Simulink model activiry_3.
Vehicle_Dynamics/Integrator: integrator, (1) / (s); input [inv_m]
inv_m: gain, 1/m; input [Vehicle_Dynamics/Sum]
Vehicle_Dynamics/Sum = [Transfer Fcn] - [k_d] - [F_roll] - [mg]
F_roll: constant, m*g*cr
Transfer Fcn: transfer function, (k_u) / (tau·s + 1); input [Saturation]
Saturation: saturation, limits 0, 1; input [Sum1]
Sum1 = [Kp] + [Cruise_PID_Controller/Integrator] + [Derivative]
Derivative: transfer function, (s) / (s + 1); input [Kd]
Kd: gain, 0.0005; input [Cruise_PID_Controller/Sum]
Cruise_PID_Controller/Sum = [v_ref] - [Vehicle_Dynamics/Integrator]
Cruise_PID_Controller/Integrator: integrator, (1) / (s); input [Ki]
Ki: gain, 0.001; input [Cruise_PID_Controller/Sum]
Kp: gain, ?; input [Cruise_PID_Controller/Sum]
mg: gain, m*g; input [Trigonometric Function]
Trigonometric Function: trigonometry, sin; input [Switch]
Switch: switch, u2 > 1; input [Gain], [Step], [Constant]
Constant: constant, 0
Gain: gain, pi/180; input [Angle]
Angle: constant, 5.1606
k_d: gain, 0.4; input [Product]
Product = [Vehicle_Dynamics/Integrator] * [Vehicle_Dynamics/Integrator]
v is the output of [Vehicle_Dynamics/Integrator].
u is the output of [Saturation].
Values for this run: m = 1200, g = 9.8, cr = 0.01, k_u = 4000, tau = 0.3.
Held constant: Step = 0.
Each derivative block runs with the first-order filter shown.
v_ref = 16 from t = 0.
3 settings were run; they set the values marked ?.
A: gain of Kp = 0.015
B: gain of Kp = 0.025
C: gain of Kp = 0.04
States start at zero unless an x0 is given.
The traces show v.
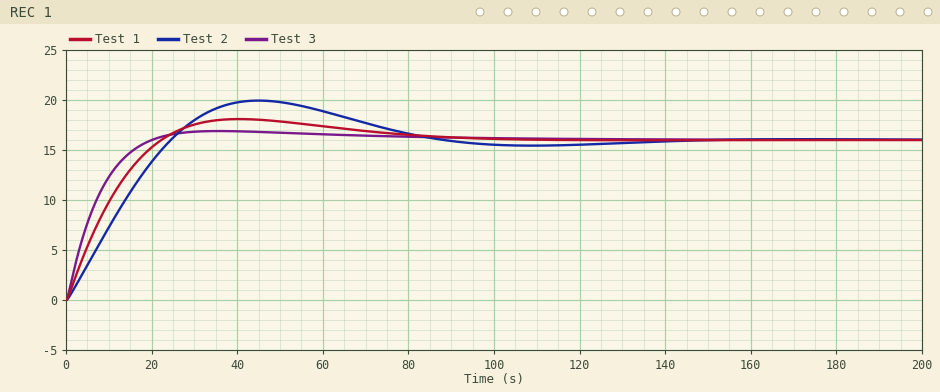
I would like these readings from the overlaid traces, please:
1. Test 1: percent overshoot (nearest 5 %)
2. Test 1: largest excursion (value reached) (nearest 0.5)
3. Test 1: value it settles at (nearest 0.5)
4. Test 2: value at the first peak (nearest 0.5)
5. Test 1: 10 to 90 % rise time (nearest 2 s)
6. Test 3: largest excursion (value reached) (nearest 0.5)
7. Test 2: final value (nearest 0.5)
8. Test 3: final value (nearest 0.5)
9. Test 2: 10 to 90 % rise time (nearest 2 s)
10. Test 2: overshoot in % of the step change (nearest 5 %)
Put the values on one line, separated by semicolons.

15 %; 18.0; 16.0; 20.0; 16 s; 17.0; 16.0; 16.0; 18 s; 25 %
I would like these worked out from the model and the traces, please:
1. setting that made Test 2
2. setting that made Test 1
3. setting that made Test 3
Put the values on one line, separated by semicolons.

A; B; C
